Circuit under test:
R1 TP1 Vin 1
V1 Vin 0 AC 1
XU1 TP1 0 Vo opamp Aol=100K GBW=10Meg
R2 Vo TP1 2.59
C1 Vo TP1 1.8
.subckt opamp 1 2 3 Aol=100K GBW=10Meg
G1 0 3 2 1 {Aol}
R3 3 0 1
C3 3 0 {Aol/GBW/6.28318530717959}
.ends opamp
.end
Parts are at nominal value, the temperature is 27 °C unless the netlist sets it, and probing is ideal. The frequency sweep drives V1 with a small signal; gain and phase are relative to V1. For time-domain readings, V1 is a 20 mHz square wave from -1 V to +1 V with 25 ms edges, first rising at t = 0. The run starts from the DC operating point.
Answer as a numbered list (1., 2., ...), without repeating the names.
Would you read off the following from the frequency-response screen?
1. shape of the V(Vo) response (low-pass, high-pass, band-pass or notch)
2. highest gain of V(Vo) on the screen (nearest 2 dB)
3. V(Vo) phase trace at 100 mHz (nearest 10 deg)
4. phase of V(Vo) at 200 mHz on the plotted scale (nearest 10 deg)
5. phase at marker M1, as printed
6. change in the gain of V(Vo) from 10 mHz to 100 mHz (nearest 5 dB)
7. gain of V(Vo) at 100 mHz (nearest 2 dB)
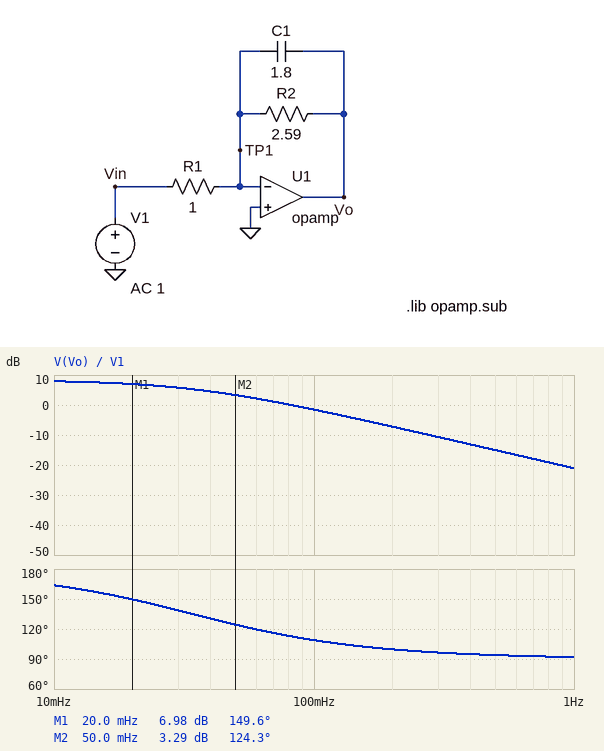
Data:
1. low-pass
2. 8 dB
3. 110 deg
4. 100 deg
5. 149.6 deg
6. -10 dB
7. -2 dB
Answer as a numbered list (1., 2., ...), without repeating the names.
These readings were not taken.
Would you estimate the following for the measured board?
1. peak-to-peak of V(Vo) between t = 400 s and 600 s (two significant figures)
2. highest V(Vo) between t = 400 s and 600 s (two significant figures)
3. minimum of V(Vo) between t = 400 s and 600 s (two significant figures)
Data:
1. 5.1 V
2. 2.6 V
3. -2.6 V
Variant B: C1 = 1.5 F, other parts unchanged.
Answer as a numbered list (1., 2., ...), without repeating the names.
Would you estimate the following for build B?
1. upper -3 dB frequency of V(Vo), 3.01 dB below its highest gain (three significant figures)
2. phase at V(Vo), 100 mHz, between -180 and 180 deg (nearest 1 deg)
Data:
1. 41.0 mHz
2. 112 deg
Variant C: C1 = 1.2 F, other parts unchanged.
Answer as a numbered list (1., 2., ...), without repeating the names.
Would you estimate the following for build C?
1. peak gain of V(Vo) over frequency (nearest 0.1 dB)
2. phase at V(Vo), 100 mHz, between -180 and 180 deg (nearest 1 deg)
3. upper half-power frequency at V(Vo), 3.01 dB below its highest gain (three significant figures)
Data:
1. 8.3 dB
2. 117 deg
3. 51.2 mHz
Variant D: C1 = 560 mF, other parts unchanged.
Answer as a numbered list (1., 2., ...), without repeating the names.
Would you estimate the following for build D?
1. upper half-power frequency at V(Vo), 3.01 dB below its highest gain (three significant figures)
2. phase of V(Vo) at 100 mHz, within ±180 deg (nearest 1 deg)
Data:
1. 110 mHz
2. 138 deg
